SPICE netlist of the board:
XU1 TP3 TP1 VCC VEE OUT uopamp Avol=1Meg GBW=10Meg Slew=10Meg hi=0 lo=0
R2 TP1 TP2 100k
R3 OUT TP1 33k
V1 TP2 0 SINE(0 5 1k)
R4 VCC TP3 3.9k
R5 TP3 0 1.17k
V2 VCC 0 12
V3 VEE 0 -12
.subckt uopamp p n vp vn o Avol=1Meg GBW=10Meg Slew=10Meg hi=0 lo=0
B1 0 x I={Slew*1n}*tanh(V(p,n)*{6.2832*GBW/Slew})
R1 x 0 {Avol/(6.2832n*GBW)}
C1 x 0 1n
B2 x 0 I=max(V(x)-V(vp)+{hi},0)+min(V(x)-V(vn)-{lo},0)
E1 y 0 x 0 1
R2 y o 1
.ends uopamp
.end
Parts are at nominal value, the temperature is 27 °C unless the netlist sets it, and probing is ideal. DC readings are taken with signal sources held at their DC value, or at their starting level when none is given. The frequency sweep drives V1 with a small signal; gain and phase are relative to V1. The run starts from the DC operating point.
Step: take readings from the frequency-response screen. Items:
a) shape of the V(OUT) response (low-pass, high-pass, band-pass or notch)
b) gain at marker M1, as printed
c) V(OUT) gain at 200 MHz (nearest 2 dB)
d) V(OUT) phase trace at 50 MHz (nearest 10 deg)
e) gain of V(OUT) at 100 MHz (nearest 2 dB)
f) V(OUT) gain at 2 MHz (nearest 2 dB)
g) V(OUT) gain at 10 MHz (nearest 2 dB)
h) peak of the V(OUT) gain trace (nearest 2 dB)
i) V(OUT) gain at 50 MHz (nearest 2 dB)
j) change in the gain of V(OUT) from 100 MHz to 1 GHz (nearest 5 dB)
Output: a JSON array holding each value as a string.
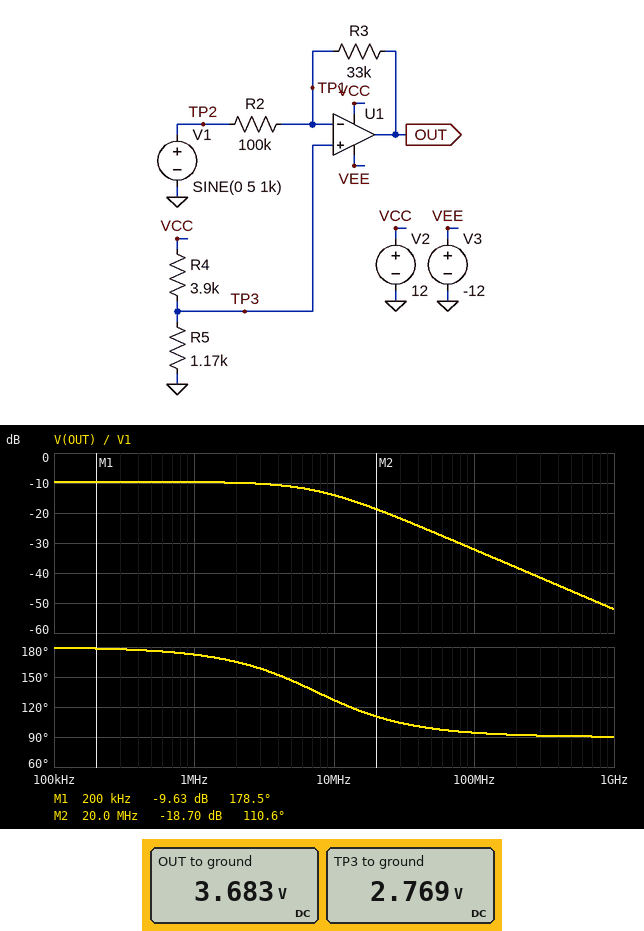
["low-pass", "-9.63 dB", "-38 dB", "100 deg", "-32 dB", "-10 dB", "-14 dB", "-10 dB", "-26 dB", "-20 dB"]
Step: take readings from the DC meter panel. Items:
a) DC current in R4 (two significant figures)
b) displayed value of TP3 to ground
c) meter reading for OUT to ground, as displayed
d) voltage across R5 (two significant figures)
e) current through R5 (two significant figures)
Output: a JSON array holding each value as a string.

["2.4 mA", "2.769 V", "3.683 V", "2.8 V", "2.4 mA"]
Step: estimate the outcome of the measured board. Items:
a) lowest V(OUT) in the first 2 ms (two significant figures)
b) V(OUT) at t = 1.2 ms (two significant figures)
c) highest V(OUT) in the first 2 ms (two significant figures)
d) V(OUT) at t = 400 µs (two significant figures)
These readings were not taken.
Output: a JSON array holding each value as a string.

["2.0 V", "2.1 V", "5.3 V", "2.7 V"]
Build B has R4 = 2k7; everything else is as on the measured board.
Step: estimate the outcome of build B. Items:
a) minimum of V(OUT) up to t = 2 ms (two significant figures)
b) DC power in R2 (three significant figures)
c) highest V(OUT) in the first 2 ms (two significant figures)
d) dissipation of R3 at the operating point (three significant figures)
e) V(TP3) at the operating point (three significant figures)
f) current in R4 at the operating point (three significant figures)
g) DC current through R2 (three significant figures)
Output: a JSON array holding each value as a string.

["3.2 V", "132 µW", "6.5 V", "43.4 µW", "3.63 V", "3.10 mA", "36.3 µA"]
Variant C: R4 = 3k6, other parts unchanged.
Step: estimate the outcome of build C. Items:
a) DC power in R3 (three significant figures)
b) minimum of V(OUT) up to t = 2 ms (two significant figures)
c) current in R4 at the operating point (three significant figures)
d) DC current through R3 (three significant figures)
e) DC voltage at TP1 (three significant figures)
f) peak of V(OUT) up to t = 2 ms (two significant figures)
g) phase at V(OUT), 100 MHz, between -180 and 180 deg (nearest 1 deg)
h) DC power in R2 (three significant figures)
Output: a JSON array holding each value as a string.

["28.6 µW", "2.3 V", "2.52 mA", "29.4 µA", "2.94 V", "5.6 V", "94 deg", "86.6 µW"]
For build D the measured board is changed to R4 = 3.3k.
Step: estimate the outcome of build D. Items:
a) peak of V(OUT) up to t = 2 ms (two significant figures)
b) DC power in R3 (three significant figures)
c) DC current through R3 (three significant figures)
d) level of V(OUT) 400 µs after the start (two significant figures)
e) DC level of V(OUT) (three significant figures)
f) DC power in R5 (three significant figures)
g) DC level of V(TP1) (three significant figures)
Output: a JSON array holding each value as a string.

["5.8 V", "32.6 µW", "31.4 µA", "3.2 V", "4.18 V", "8.43 mW", "3.14 V"]
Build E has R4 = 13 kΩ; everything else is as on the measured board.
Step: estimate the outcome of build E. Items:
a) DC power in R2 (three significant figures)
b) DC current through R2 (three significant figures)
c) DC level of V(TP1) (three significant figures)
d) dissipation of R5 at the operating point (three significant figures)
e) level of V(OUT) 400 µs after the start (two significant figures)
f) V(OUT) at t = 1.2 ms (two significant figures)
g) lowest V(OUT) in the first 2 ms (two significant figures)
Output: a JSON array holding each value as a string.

["9.82 µW", "9.91 µA", "991 mV", "839 µW", "350 mV", "-250 mV", "-330 mV"]
